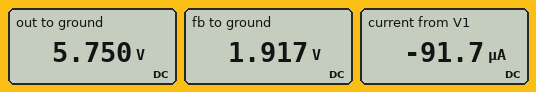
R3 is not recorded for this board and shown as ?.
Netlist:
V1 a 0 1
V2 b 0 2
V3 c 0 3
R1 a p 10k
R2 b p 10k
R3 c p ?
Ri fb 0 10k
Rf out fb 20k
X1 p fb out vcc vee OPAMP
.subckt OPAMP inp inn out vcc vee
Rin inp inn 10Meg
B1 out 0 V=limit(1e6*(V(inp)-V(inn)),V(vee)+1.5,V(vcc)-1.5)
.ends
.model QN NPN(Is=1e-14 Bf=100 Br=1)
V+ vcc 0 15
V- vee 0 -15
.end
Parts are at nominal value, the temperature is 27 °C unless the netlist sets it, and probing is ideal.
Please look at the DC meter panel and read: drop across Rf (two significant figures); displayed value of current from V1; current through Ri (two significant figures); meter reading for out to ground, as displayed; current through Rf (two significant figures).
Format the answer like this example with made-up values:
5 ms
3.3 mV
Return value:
3.8 V
-91.7 µA
190 µA
5.750 V
190 µA
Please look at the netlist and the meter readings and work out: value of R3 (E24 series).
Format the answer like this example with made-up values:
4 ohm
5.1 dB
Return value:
13 kΩ
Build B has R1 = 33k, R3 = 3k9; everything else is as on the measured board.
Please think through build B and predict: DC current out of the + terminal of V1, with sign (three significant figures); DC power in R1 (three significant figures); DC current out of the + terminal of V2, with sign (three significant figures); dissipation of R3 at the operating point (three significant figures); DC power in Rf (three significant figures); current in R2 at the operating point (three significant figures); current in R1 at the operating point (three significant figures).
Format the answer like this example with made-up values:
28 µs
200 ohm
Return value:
-48.0 µA
76.1 µW
-58.5 µA
44.2 µW
1.34 mW
58.5 µA
48.0 µA
